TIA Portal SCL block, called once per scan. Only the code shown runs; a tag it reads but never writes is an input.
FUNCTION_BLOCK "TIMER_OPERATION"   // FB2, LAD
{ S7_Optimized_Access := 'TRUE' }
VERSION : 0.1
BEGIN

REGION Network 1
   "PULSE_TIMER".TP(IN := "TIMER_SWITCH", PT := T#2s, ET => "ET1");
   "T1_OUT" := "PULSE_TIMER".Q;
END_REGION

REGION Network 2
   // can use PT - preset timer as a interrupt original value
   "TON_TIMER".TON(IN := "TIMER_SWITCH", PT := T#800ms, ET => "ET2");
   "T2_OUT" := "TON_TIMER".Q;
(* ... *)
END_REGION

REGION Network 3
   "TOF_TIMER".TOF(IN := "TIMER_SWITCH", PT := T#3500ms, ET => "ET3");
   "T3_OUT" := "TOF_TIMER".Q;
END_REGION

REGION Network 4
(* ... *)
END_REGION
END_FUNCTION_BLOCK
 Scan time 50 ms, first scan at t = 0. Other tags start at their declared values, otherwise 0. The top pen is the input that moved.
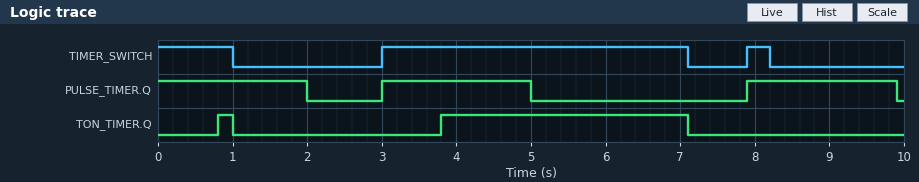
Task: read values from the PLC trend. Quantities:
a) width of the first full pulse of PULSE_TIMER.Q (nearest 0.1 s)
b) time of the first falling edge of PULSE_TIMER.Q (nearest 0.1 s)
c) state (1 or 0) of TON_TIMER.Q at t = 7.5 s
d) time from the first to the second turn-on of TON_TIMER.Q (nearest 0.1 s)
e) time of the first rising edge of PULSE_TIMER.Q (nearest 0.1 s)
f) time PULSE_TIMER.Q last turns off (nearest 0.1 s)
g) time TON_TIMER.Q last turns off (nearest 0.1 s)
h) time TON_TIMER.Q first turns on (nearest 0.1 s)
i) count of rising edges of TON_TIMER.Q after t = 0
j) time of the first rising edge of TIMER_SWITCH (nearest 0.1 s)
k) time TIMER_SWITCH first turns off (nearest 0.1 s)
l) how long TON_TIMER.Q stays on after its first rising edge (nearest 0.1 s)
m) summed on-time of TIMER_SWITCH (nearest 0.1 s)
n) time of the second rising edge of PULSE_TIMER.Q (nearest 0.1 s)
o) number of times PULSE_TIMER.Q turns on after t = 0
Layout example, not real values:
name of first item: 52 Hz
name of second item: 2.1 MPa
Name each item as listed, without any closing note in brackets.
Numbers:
width of the first full pulse of PULSE_TIMER.Q: 2.0 s
time of the first falling edge of PULSE_TIMER.Q: 2.0 s
state (1 or 0) of TON_TIMER.Q at t = 7.5 s: 0
time from the first to the second turn-on of TON_TIMER.Q: 3.0 s
time of the first rising edge of PULSE_TIMER.Q: 3.0 s
time PULSE_TIMER.Q last turns off: 9.9 s
time TON_TIMER.Q last turns off: 7.1 s
time TON_TIMER.Q first turns on: 0.8 s
count of rising edges of TON_TIMER.Q after t = 0: 2
time of the first rising edge of TIMER_SWITCH: 3.0 s
time TIMER_SWITCH first turns off: 1.0 s
how long TON_TIMER.Q stays on after its first rising edge: 0.2 s
summed on-time of TIMER_SWITCH: 5.4 s
time of the second rising edge of PULSE_TIMER.Q: 7.9 s
number of times PULSE_TIMER.Q turns on after t = 0: 2
